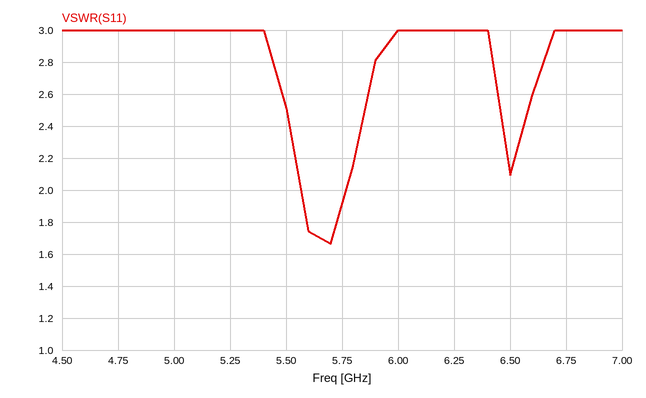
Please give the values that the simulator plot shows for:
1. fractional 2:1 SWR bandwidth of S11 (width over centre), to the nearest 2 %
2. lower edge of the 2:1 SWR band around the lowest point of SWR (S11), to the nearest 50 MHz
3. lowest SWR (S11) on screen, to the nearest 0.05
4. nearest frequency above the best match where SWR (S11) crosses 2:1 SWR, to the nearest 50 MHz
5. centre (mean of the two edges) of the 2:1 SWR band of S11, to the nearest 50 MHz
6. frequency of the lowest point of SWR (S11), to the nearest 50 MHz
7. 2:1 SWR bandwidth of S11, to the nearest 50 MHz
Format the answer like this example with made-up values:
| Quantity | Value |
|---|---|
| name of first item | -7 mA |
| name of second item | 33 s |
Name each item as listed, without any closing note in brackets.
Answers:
| Quantity | Value |
|---|---|
| fractional 2:1 SWR bandwidth of S11 (width over centre), to the nearest 2 % | 4 % |
| lower edge of the 2:1 SWR band around the lowest point of SWR (S11), to the nearest 50 MHz | 5.55 GHz |
| lowest SWR (S11) on screen, to the nearest 0.05 | 1.65 |
| nearest frequency above the best match where SWR (S11) crosses 2:1 SWR, to the nearest 50 MHz | 5.75 GHz |
| centre (mean of the two edges) of the 2:1 SWR band of S11, to the nearest 50 MHz | 5.65 GHz |
| frequency of the lowest point of SWR (S11), to the nearest 50 MHz | 5.70 GHz |
| 2:1 SWR bandwidth of S11, to the nearest 50 MHz | 200 MHz |
